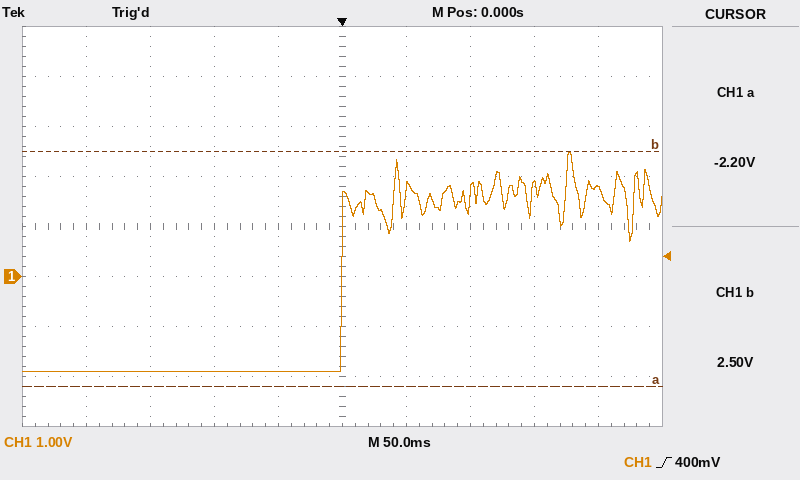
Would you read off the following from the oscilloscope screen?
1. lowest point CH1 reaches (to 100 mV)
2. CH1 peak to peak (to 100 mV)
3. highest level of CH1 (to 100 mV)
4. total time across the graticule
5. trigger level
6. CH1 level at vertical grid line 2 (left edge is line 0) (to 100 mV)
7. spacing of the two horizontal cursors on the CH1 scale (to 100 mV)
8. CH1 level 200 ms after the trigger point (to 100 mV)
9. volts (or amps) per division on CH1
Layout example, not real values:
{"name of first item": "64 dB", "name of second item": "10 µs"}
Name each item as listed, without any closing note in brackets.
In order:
{"lowest point CH1 reaches": "-1.9 V", "CH1 peak to peak": "4.4 V", "highest level of CH1": "2.5 V", "total time across the graticule": "500 ms", "trigger level": "400 mV", "CH1 level at vertical grid line 2 (left edge is line 0)": "-1.9 V", "spacing of the two horizontal cursors on the CH1 scale": "4.7 V", "CH1 level 200 ms after the trigger point": "1.8 V", "volts (or amps) per division on CH1": "1 V"}
